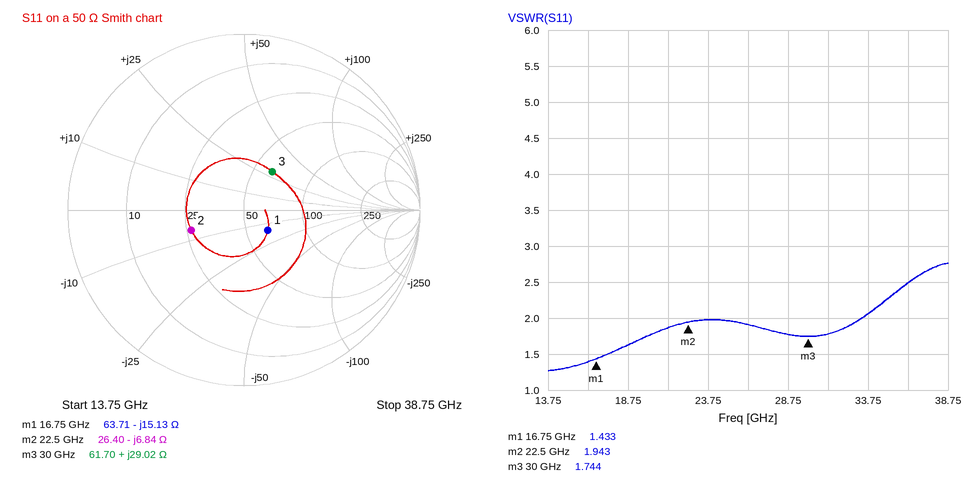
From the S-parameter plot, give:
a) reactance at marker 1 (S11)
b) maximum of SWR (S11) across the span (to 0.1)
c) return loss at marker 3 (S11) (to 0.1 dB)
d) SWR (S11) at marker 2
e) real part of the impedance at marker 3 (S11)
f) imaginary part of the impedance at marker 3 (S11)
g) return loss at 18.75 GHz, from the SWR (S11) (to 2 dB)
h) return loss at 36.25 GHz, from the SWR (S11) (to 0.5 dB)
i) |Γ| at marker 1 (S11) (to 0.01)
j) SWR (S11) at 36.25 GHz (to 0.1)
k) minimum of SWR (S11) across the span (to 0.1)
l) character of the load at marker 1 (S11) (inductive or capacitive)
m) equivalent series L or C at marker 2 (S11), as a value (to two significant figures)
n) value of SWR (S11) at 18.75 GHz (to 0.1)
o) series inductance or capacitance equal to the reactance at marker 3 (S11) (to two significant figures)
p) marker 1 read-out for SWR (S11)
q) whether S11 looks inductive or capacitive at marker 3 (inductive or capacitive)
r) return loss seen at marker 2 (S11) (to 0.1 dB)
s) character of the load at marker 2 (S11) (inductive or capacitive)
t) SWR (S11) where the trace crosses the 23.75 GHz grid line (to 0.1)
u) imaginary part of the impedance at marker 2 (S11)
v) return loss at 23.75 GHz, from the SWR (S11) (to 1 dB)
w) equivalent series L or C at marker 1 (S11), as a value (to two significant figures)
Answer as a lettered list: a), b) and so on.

a) -15.13 Ω
b) 2.8
c) 11.3 dB
d) 1.943
e) 61.70 Ω
f) +29.02 Ω
g) 12 dB
h) 7.5 dB
i) 0.18
j) 2.5
k) 1.3
l) capacitive
m) 1.0 pF
n) 1.6
o) 150 pH
p) 1.433
q) inductive
r) 9.9 dB
s) capacitive
t) 2.0
u) -6.84 Ω
v) 10 dB
w) 630 fF
